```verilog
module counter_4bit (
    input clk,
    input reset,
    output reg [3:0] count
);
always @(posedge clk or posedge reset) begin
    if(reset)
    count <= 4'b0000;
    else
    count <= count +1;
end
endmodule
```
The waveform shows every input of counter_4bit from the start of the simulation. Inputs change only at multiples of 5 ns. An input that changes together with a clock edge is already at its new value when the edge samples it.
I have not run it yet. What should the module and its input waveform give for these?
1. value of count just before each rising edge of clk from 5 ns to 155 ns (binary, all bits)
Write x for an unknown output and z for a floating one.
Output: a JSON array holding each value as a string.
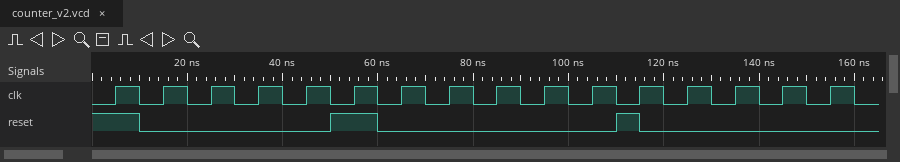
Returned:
["0000, 0000, 0001, 0010, 0011, 0000, 0000, 0001, 0010, 0011, 0100, 0000, 0001, 0010, 0011, 0100"]
